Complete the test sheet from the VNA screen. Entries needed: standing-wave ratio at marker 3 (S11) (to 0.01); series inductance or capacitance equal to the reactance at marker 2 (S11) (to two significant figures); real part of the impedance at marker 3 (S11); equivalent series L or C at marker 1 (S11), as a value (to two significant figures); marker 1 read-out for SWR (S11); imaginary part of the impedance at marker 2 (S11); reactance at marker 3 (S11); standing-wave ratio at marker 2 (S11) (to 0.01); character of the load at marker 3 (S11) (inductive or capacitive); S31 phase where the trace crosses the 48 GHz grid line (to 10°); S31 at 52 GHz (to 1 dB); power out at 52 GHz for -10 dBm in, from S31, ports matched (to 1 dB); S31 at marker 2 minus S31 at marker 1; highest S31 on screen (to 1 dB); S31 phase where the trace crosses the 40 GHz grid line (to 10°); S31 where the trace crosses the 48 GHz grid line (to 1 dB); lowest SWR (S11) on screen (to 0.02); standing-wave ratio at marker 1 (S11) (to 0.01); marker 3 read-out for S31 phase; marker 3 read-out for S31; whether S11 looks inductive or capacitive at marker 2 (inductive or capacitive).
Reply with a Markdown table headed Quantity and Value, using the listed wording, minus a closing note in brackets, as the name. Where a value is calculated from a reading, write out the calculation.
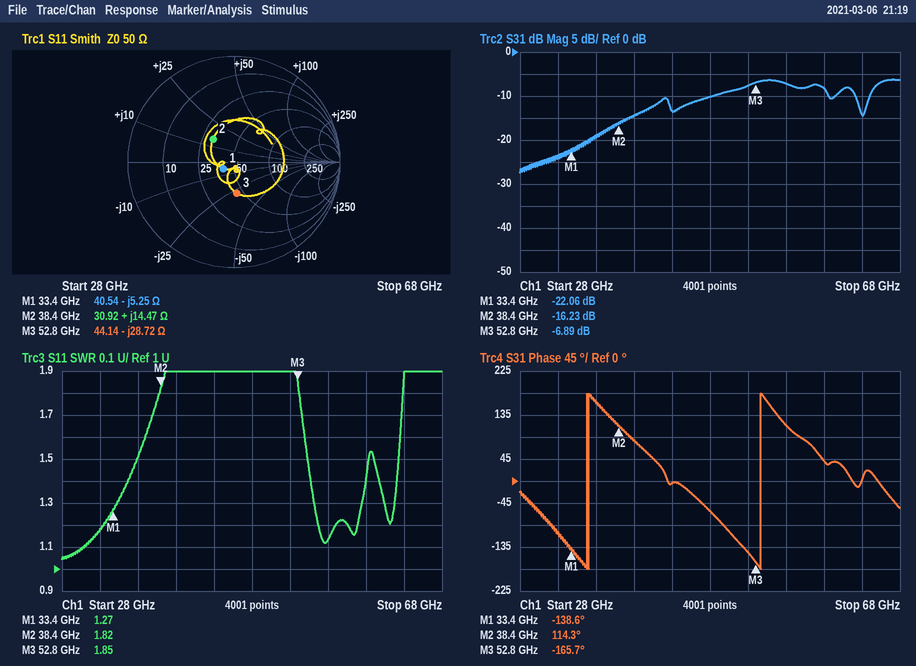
| Quantity | Value |
|---|---|
| standing-wave ratio at marker 3 (S11) | 1.85 |
| series inductance or capacitance equal to the reactance at marker 2 (S11) | L = 14.47 Ω/(2π × 38.4 GHz) ≈ 60 pH |
| real part of the impedance at marker 3 | 44.14 Ω |
| equivalent series L or C at marker 1 (S11), as a value | C = 1/(2π × 33.4 GHz × 5.25 Ω) ≈ 908 fF, so 910 fF to two significant figures |
| marker 1 read-out for SWR | 1.27 |
| imaginary part of the impedance at marker 2 | +14.47 Ω |
| reactance at marker 3 | -28.72 Ω |
| standing-wave ratio at marker 2 (S11) | 1.82 |
| character of the load at marker 3 (S11) | capacitive |
| S31 phase where the trace crosses the 48 GHz grid line | -60° |
| S31 at 52 GHz | -8 dB |
| power out at 52 GHz for -10 dBm in, from S31, ports matched | -10 dBm + (-8 dB) = -18 dBm |
| S31 at marker 2 minus S31 at marker 1 | -16.23 − (-22.06) = 5.83 dB |
| highest S31 on screen | -6 dB |
| S31 phase where the trace crosses the 40 GHz grid line | 80° |
| S31 where the trace crosses the 48 GHz grid line | -10 dB |
| lowest SWR (S11) on screen | 1.04 |
| standing-wave ratio at marker 1 (S11) | 1.27 |
| marker 3 read-out for S31 phase | -165.7° |
| marker 3 read-out for S31 | -6.89 dB |
| whether S11 looks inductive or capacitive at marker 2 | inductive |
